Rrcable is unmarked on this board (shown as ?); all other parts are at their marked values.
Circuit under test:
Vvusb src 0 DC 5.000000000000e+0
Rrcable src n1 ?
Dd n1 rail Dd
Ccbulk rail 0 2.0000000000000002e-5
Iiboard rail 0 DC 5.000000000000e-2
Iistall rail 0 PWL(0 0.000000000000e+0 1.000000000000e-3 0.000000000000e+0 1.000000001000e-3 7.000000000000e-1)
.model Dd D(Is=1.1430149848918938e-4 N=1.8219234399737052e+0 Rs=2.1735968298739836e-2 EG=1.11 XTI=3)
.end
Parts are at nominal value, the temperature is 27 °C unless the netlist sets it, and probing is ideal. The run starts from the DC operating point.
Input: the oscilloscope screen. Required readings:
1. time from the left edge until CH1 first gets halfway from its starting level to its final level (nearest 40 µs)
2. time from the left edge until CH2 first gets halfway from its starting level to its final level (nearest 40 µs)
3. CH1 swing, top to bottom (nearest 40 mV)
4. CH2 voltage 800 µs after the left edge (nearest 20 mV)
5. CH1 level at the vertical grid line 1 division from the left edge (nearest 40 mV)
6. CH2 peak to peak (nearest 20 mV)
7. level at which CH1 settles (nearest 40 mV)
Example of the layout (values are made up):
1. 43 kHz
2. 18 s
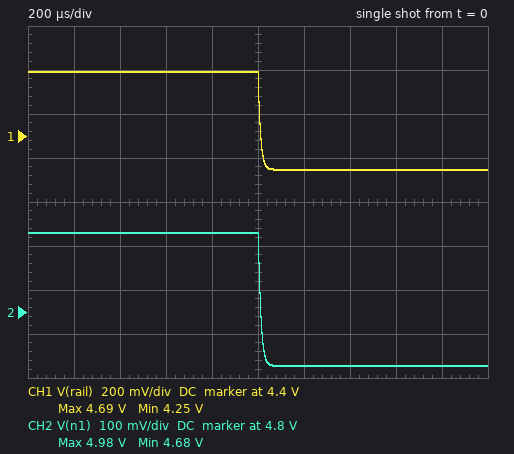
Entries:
1. 1.00 ms
2. 1.00 ms
3. 440 mV
4. 4.98 V
5. 4.68 V
6. 300 mV
7. 4.24 V
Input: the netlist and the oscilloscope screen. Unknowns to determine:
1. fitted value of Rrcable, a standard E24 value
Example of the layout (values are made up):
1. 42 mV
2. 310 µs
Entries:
1. 0.43 Ω
